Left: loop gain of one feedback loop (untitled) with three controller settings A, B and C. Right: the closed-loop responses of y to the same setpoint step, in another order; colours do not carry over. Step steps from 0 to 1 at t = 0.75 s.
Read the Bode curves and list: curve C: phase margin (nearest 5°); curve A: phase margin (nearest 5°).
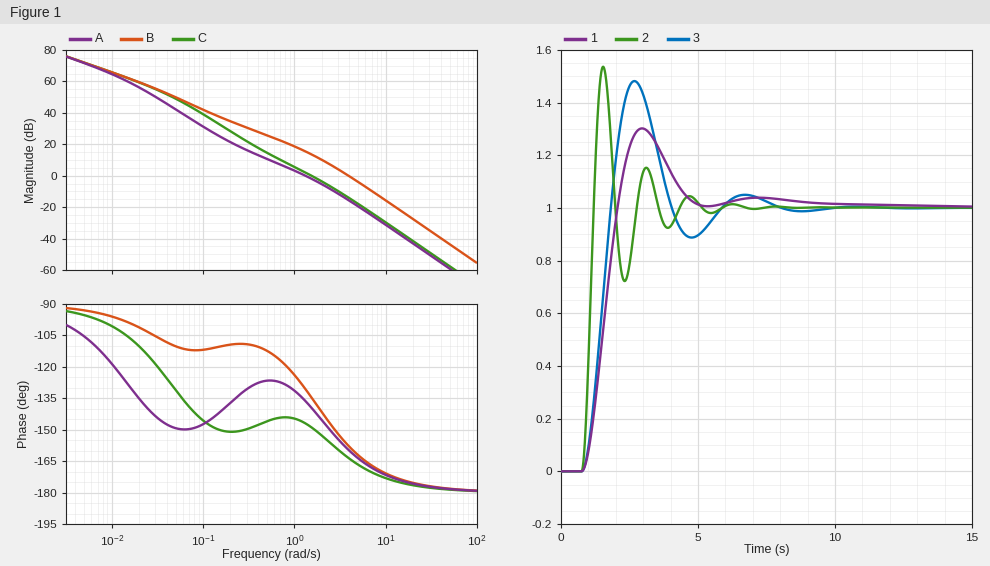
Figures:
30°
45°
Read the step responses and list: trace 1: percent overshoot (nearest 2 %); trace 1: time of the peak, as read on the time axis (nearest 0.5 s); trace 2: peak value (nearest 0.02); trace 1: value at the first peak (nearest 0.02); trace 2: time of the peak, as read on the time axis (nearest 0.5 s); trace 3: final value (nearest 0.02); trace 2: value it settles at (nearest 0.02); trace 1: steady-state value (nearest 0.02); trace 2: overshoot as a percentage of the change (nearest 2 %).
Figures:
30 %
3.0 s
1.54
1.30
1.5 s
1.00
1.00
1.00
54 %
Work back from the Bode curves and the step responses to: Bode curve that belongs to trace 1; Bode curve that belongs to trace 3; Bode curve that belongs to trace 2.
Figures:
A
C
B
